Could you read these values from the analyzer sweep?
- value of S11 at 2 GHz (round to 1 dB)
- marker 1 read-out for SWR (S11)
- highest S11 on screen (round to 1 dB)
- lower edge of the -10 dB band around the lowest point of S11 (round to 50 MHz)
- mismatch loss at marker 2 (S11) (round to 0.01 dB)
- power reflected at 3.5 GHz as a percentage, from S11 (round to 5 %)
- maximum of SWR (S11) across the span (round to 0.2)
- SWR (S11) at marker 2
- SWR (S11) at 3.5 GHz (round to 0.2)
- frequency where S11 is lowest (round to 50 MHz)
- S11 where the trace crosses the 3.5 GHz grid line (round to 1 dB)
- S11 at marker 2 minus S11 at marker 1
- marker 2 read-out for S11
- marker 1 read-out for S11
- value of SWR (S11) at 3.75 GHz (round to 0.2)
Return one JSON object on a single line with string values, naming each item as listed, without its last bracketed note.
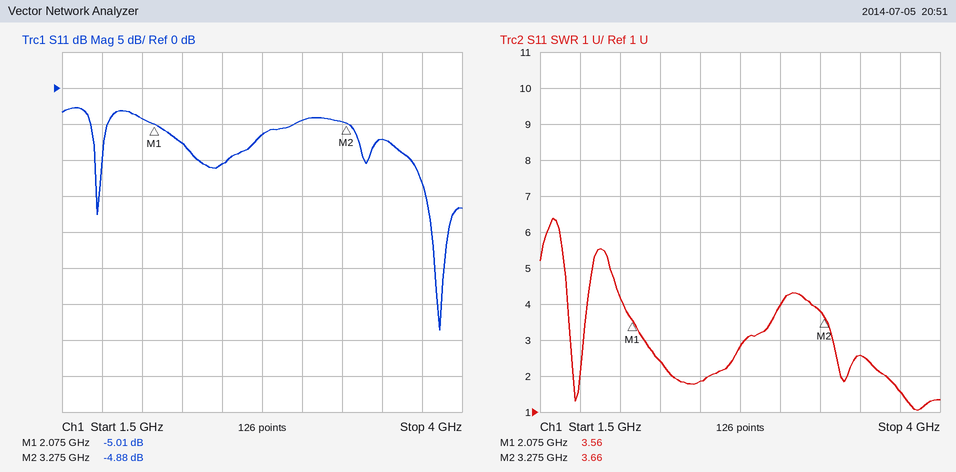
{"value of S11 at 2 GHz": "-4 dB", "marker 1 read-out for SWR": "3.56", "highest S11 on screen": "-3 dB", "lower edge of the -10 dB band around the lowest point of S11": "3.70 GHz", "mismatch loss at marker 2 (S11)": "1.71 dB", "power reflected at 3.5 GHz as a percentage, from S11": "20 %", "maximum of SWR (S11) across the span": "6.4", "SWR (S11) at marker 2": "3.66", "SWR (S11) at 3.5 GHz": "2.6", "frequency where S11 is lowest": "3.85 GHz", "S11 where the trace crosses the 3.5 GHz grid line": "-7 dB", "S11 at marker 2 minus S11 at marker 1": "0.13 dB", "marker 2 read-out for S11": "-4.88 dB", "marker 1 read-out for S11": "-5.01 dB", "value of SWR (S11) at 3.75 GHz": "1.6"}
